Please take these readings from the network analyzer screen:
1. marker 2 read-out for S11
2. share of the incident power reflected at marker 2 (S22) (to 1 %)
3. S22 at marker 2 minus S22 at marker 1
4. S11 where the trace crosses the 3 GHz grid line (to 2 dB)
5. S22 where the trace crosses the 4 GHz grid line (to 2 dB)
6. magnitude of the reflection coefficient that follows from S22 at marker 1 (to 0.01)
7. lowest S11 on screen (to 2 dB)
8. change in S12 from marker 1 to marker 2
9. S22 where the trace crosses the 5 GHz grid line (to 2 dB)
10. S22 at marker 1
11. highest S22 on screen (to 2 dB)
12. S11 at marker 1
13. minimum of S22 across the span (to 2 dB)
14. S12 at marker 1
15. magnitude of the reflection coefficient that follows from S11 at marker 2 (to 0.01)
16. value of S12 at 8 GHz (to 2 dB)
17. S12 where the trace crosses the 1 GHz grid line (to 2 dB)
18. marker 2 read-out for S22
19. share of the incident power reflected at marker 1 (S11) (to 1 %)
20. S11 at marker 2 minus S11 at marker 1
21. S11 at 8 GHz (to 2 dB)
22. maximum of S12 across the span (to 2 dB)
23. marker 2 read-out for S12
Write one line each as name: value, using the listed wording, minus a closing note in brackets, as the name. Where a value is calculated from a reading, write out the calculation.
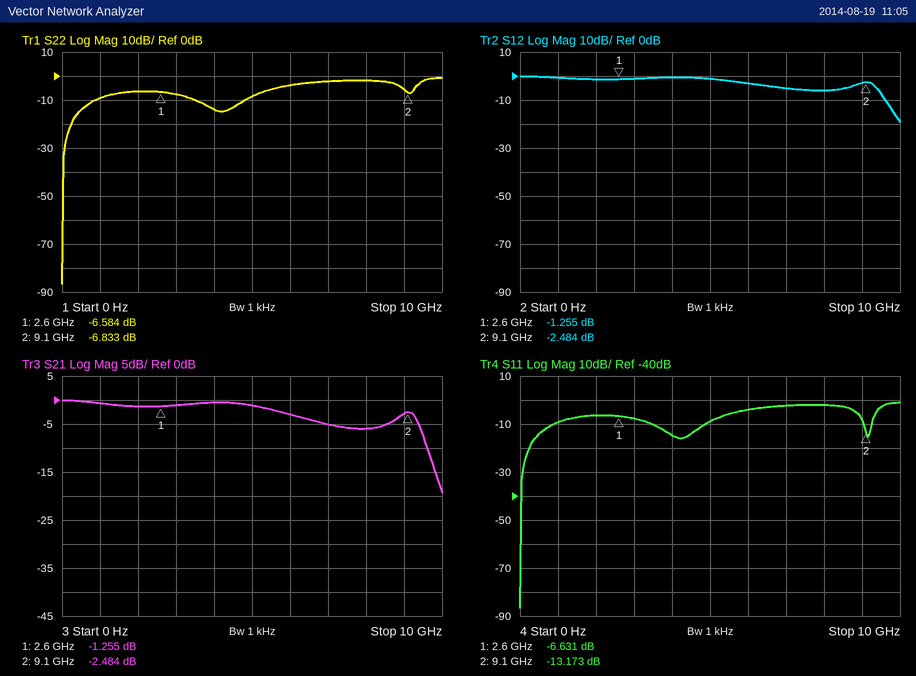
marker 2 read-out for S11: -13.173 dB
share of the incident power reflected at marker 2 (S22): 10^(-6.833/10) ≈ 21 %
S22 at marker 2 minus S22 at marker 1: -6.833 − (-6.584) = -0.249 dB
S11 where the trace crosses the 3 GHz grid line: -8 dB
S22 where the trace crosses the 4 GHz grid line: -14 dB
magnitude of the reflection coefficient that follows from S22 at marker 1: 10^(-6.584/20) ≈ 0.47
lowest S11 on screen: -86 dB
change in S12 from marker 1 to marker 2: -2.484 − (-1.255) = -1.229 dB
S22 where the trace crosses the 5 GHz grid line: -8 dB
S22 at marker 1: -6.584 dB
highest S22 on screen: 0 dB
S11 at marker 1: -6.631 dB
minimum of S22 across the span: -86 dB
S12 at marker 1: -1.255 dB
magnitude of the reflection coefficient that follows from S11 at marker 2: 10^(-13.173/20) ≈ 0.22
value of S12 at 8 GHz: -6 dB
S12 where the trace crosses the 1 GHz grid line: 0 dB
marker 2 read-out for S22: -6.833 dB
share of the incident power reflected at marker 1 (S11): 10^(-6.631/10) ≈ 22 %
S11 at marker 2 minus S11 at marker 1: -13.173 − (-6.631) = -6.542 dB
S11 at 8 GHz: -2 dB
maximum of S12 across the span: 0 dB
marker 2 read-out for S12: -2.484 dB
